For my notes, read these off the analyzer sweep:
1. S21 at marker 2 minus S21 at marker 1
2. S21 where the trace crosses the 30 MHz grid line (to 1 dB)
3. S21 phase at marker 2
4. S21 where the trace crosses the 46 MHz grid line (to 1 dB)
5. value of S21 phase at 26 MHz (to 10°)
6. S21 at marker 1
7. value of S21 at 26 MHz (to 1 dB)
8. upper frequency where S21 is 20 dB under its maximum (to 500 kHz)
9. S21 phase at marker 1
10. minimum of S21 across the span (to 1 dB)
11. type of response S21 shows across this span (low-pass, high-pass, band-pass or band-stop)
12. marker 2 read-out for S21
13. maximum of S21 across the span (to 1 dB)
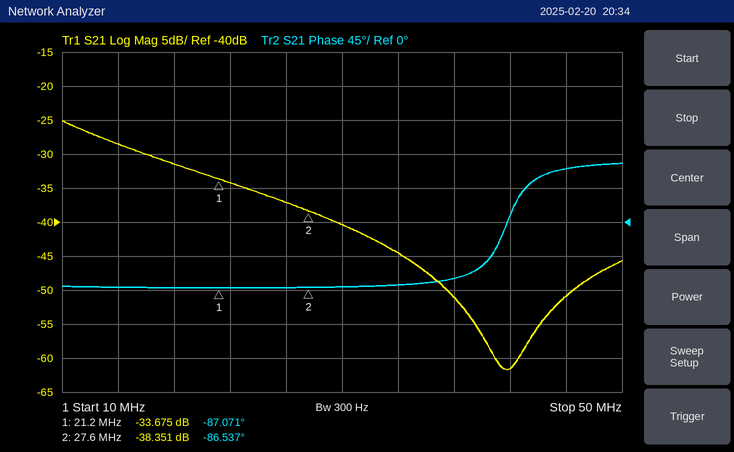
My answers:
-4.676 dB
-40 dB
-86.537°
-51 dB
-90°
-33.675 dB
-37 dB
34.5 MHz
-87.071°
-62 dB
low-pass
-38.351 dB
-25 dB
